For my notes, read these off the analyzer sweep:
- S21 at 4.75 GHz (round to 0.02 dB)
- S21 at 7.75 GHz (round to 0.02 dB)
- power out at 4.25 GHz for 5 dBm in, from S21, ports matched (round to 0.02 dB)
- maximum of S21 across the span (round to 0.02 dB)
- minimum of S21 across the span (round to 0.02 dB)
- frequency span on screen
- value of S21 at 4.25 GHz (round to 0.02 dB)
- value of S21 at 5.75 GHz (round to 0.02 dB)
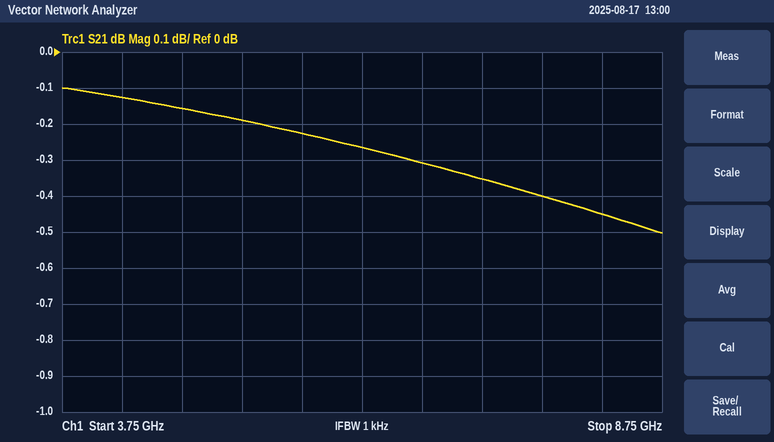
-0.16 dB
-0.40 dB
4.88 dBm
-0.10 dB
-0.50 dB
5 GHz
-0.12 dB
-0.22 dB
